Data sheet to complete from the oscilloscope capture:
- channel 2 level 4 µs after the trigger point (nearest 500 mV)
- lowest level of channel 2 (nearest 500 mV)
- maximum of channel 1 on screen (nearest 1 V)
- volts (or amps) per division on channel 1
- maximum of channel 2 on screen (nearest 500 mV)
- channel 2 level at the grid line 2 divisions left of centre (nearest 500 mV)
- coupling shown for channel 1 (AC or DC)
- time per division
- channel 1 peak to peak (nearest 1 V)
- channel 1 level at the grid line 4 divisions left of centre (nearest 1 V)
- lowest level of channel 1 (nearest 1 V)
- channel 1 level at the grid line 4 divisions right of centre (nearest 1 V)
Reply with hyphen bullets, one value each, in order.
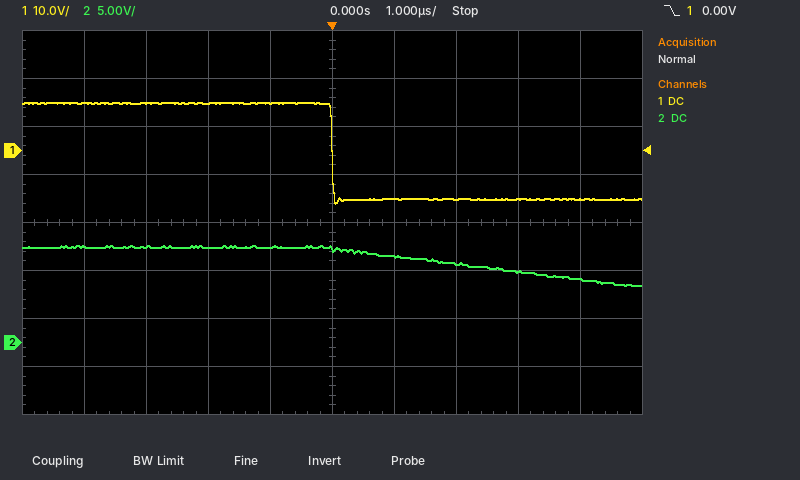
- 6.5 V
- 6.0 V
- 10 V
- 10 V
- 10.0 V
- 10.0 V
- DC
- 1 µs
- 21 V
- 10 V
- -11 V
- -10 V
